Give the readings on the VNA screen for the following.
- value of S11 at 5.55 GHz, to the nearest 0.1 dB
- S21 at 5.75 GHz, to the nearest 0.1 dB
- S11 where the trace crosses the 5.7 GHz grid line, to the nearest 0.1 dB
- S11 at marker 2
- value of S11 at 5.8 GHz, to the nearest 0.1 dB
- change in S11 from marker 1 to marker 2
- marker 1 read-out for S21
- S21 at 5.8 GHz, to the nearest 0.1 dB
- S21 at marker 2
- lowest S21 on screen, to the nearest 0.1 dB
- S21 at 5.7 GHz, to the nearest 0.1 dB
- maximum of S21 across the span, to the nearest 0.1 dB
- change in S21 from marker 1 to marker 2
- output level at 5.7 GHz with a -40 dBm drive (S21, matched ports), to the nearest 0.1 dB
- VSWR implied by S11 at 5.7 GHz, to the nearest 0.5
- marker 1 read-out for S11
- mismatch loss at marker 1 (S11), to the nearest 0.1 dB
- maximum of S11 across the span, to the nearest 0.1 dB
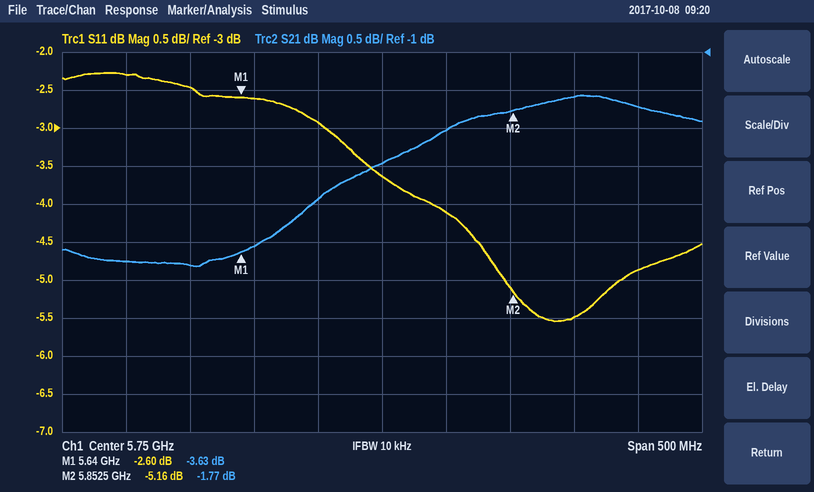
-2.3 dB
-2.5 dB
-2.9 dB
-5.16 dB
-4.1 dB
-2.56 dB
-3.63 dB
-2.0 dB
-1.77 dB
-3.8 dB
-2.9 dB
-1.6 dB
1.86 dB
-42.9 dBm
6.0
-2.60 dB
3.5 dB
-2.3 dB
